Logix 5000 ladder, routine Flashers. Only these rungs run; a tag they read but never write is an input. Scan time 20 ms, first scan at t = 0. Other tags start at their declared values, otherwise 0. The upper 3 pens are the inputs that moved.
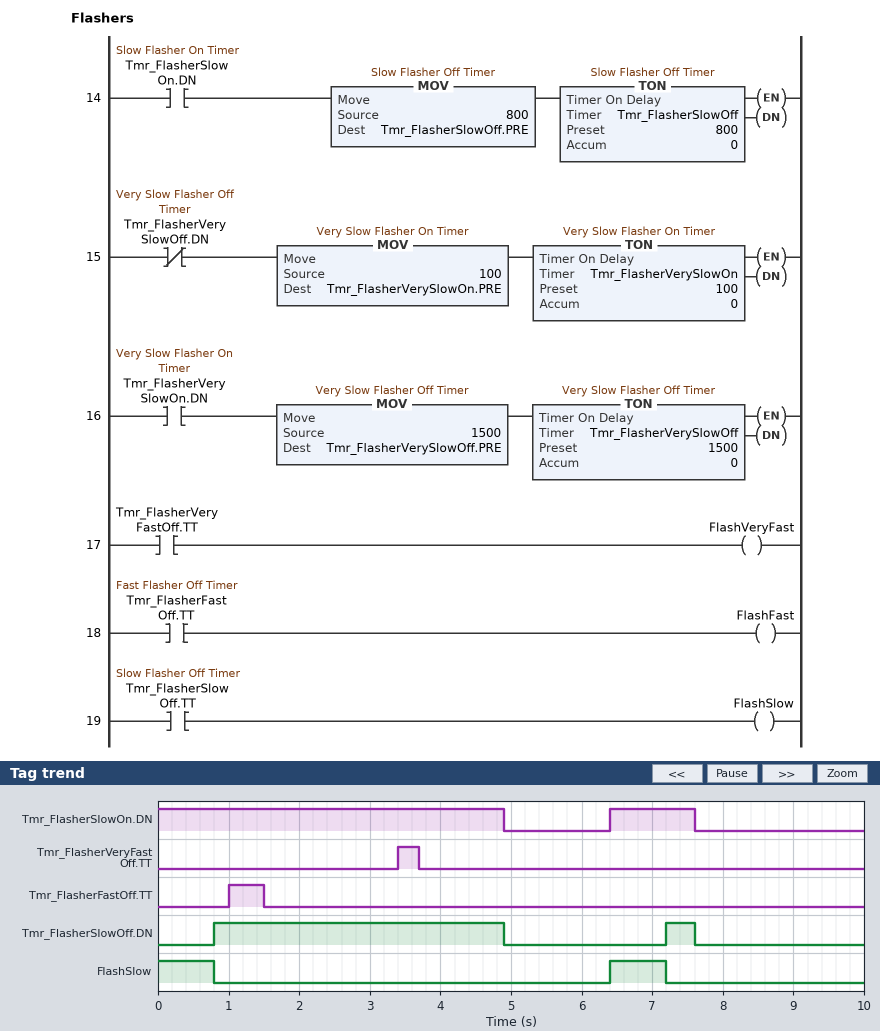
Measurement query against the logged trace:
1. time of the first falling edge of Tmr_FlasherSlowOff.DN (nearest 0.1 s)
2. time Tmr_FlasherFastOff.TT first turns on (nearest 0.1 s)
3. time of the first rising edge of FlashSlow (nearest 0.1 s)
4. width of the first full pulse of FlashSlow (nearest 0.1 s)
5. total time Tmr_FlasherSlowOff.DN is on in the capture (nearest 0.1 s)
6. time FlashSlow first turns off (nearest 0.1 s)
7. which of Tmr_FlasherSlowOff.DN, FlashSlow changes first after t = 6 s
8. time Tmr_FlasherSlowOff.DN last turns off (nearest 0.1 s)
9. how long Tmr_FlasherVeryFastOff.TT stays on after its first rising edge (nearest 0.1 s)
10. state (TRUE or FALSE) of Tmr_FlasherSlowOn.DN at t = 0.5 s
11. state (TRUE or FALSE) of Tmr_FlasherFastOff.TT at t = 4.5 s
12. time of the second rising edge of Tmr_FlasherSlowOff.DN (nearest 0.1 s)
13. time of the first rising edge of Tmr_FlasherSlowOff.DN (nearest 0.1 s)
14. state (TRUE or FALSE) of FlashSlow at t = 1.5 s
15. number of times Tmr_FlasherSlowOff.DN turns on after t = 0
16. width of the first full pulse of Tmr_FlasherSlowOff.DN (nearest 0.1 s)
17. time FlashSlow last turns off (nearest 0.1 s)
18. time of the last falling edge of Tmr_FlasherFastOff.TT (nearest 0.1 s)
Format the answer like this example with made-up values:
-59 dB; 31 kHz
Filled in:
4.9 s; 1.0 s; 6.4 s; 0.8 s; 4.5 s; 0.8 s; FlashSlow; 7.6 s; 0.3 s; TRUE; FALSE; 7.2 s; 0.8 s; FALSE; 2; 4.1 s; 7.2 s; 1.5 s
